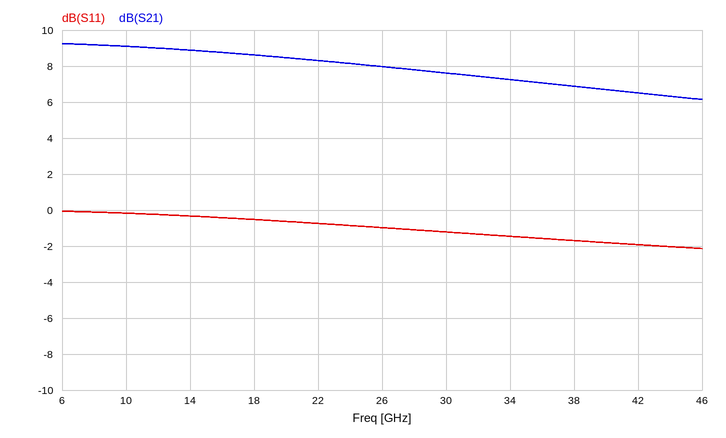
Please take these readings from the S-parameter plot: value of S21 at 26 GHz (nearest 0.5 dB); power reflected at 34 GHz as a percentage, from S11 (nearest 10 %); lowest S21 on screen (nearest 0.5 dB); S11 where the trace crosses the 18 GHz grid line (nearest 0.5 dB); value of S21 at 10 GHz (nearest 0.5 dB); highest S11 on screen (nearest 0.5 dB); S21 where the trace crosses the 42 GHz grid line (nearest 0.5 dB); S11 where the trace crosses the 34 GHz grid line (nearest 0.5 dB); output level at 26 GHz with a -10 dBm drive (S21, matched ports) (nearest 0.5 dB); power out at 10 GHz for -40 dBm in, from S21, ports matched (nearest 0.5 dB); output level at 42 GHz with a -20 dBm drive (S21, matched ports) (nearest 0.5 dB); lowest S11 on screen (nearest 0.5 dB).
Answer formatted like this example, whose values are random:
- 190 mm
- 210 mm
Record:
- 8.0 dB
- 70 %
- 6.0 dB
- -0.5 dB
- 9.0 dB
- 0.0 dB
- 6.5 dB
- -1.5 dB
- -2.0 dBm
- -31.0 dBm
- -13.5 dBm
- -2.0 dB
